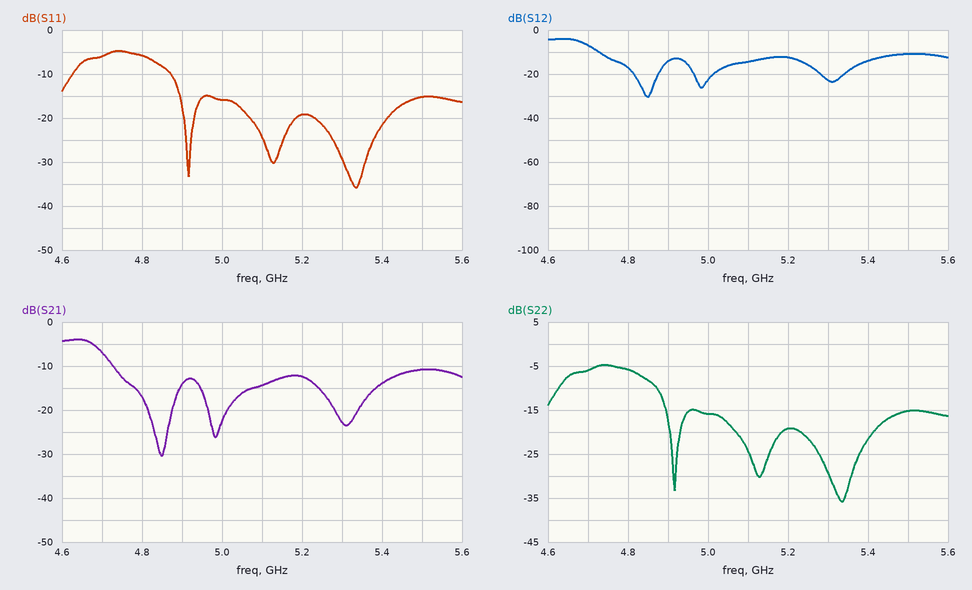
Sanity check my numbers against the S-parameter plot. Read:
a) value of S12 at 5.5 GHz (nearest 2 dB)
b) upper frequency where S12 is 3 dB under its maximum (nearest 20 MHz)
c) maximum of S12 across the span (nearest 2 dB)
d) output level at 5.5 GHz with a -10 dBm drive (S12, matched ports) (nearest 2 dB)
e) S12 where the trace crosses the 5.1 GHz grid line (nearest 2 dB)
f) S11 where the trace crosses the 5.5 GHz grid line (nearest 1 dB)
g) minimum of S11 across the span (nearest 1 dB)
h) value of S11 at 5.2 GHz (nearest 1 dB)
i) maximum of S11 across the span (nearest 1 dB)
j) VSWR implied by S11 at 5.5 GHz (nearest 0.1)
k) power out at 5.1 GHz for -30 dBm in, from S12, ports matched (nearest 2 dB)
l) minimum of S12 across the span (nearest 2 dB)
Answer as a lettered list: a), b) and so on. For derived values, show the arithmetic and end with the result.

a) -10 dB
b) 4.70 GHz
c) -4 dB
d) -10 dBm + (-10 dB) = -20 dBm
e) -14 dB
f) -15 dB
g) -36 dB
h) -19 dB
i) -5 dB
j) |Γ| = 10^(-15/20) = 0.1778; VSWR = (1 + 0.1778)/(1 − 0.1778) ≈ 1.4
k) -30 dBm + (-14 dB) = -44 dBm
l) -30 dB
